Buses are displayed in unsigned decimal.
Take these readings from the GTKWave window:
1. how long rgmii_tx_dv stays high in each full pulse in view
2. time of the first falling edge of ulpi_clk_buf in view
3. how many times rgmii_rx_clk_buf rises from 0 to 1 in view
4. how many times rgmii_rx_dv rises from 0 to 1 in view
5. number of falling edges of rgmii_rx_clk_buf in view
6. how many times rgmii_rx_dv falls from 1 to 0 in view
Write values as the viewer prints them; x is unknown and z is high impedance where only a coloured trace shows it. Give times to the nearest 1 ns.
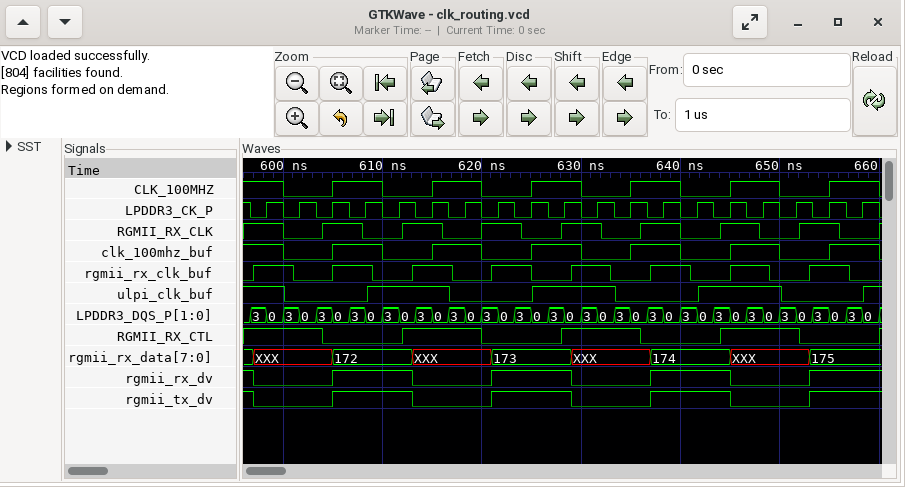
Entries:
8 ns, 8 ns, 8 ns
600 ns
8
4
8
4
